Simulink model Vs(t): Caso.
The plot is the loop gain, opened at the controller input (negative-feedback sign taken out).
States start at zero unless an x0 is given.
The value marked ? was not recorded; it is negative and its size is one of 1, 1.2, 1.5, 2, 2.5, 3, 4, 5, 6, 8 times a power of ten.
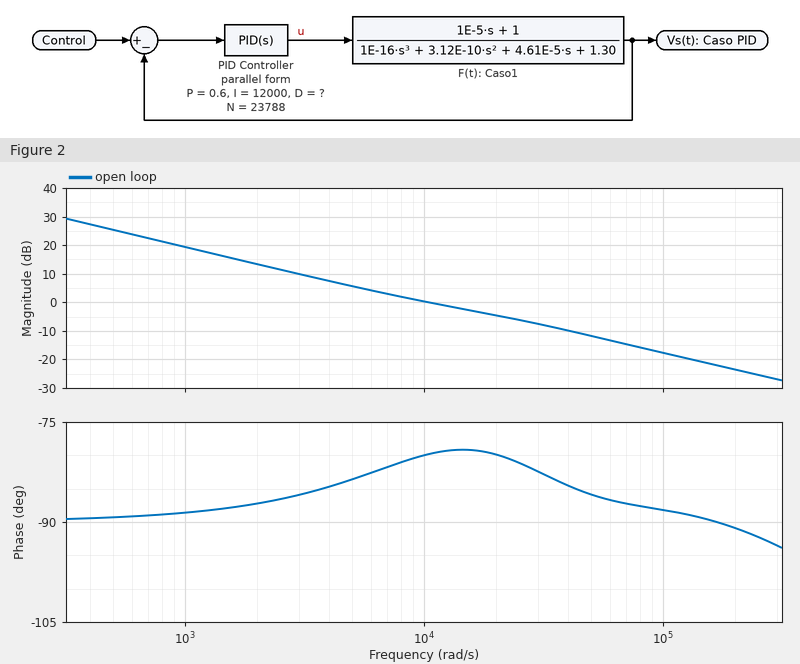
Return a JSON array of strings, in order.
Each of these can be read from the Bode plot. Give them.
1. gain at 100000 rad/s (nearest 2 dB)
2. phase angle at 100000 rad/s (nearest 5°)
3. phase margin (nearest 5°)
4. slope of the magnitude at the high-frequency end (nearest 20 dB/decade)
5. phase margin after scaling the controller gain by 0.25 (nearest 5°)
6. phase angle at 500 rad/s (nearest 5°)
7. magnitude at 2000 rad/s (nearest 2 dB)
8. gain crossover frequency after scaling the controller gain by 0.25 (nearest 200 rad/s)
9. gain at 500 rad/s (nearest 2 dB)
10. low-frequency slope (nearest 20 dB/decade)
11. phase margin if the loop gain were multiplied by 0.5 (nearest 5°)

["-18 dB", "-90°", "100°", "-20 dB/decade", "95°", "-90°", "14 dB", "2400 rad/s", "26 dB", "-20 dB/decade", "95°"]
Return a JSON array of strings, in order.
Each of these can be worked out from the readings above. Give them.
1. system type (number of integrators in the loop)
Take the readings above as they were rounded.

["1"]
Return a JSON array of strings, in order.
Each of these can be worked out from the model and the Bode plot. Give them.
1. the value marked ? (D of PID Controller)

["-8e-06"]
